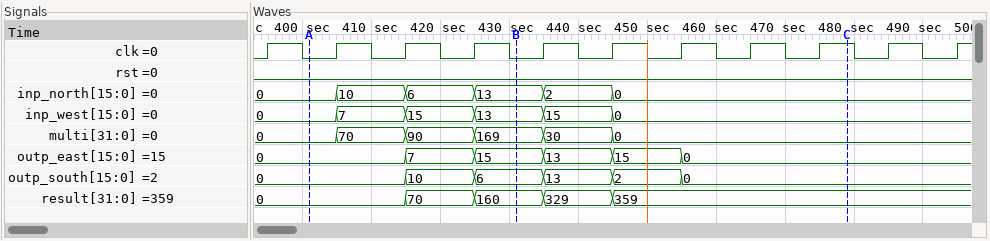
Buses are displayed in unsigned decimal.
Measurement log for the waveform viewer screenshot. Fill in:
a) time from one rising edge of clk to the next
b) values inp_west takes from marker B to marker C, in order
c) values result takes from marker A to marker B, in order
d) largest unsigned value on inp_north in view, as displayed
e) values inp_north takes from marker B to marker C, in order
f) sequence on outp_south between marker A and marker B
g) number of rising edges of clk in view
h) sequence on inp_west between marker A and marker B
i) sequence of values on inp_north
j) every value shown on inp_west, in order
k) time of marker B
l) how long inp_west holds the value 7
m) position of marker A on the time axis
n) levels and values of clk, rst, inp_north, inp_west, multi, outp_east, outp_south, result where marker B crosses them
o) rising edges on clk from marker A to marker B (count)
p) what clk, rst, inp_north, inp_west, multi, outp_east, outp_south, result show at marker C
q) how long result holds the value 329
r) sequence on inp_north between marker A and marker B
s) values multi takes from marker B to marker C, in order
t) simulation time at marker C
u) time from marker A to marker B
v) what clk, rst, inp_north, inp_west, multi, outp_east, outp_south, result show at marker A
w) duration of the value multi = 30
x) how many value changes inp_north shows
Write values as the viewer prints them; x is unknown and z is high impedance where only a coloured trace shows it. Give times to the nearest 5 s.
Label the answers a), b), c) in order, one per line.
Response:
a) 10 s
b) 13, 15, 0
c) 0, 70, 160
d) 13
e) 13, 2, 0
f) 0, 10, 6
g) 11
h) 0, 7, 15, 13
i) 0, 10, 6, 13, 2, 0
j) 0, 7, 15, 13, 15, 0
k) 430 s
l) 10 s
m) 400 s
n) clk=0, rst=0, inp_north=13, inp_west=13, multi=169, outp_east=15, outp_south=6, result=160
o) 3
p) clk=1, rst=0, inp_north=0, inp_west=0, multi=0, outp_east=0, outp_south=0, result=359
q) 10 s
r) 0, 10, 6, 13
s) 169, 30, 0
t) 480 s
u) 30 s
v) clk=0, rst=0, inp_north=0, inp_west=0, multi=0, outp_east=0, outp_south=0, result=0
w) 10 s
x) 5
